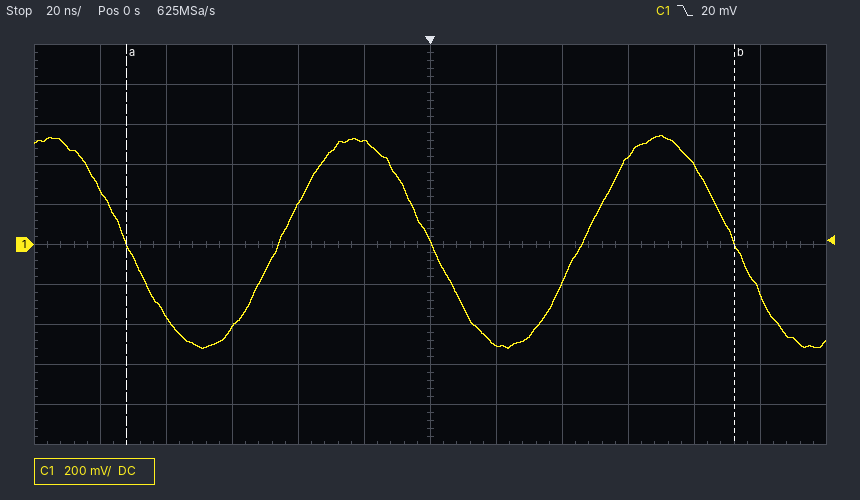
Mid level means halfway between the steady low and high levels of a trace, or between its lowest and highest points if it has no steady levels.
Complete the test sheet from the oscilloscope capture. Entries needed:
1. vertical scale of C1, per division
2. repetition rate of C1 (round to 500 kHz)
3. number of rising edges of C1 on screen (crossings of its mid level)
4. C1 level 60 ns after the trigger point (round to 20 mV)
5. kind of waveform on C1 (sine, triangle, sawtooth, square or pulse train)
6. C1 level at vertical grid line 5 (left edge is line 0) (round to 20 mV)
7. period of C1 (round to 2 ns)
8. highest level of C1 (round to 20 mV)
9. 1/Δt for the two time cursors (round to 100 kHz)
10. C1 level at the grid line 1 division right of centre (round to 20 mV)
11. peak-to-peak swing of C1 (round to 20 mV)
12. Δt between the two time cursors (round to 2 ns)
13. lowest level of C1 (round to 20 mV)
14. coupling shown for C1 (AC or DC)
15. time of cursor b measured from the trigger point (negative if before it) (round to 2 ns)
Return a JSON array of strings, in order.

["200 mV", "11.0 MHz", "2", "440 mV", "sine", "520 mV", "92 ns", "540 mV", "5.4 MHz", "-500 mV", "1.06 V", "184 ns", "-520 mV", "DC", "+92 ns"]
